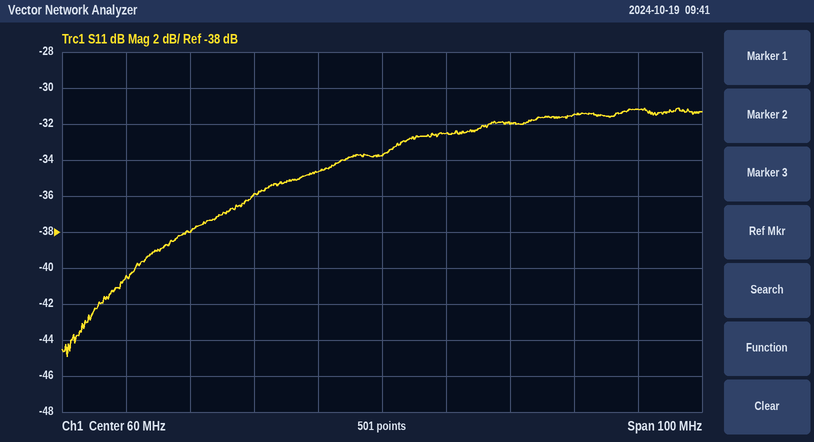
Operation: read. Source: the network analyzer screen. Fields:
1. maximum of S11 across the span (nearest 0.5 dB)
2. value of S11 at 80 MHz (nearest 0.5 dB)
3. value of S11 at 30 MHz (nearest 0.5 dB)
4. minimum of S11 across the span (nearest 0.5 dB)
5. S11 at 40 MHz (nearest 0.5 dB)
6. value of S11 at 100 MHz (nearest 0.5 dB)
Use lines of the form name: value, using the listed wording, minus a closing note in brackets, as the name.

maximum of S11 across the span: -31.0 dB
value of S11 at 80 MHz: -32.0 dB
value of S11 at 30 MHz: -38.0 dB
minimum of S11 across the span: -45.0 dB
S11 at 40 MHz: -36.0 dB
value of S11 at 100 MHz: -31.0 dB
